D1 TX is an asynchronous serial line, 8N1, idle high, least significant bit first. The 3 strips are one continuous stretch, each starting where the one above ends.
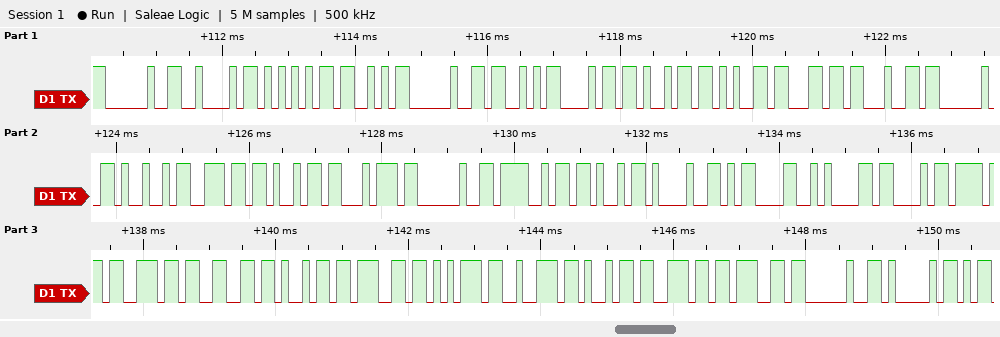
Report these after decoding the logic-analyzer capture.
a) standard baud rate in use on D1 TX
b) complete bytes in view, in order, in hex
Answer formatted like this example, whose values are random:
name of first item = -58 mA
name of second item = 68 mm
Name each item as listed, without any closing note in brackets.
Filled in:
standard baud rate in use on D1 TX = 9600 baud
complete bytes in view, in order, in hex = 20 42 55 53 20 53 68 69 65 6C 64 20 49 6E 69 74 20 4F 4B 21 0D 0A 43 6F 6E 66 69 67 75 72 69 6E 67 20 41
